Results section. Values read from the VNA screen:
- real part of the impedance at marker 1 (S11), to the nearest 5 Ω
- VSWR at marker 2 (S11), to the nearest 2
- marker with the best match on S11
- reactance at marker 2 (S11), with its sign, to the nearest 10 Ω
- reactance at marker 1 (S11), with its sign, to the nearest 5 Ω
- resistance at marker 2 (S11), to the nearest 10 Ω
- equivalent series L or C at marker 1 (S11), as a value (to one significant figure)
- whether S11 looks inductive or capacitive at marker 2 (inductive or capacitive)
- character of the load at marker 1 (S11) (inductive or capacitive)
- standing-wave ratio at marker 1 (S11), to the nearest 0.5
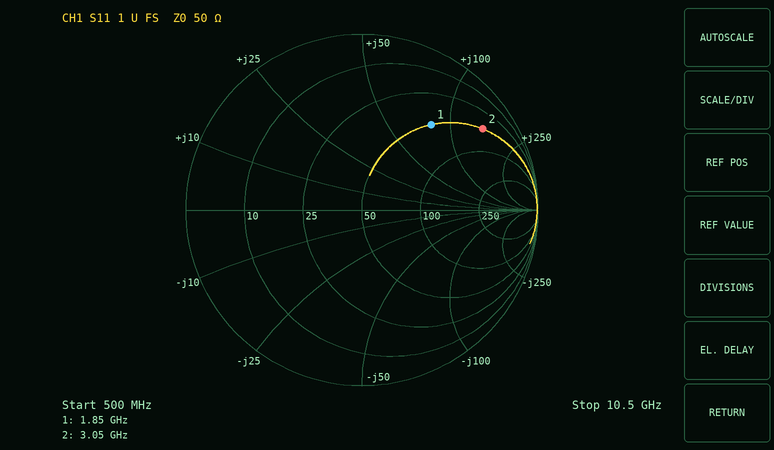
50 Ω
10
marker 1
+150 Ω
+80 Ω
50 Ω
7 nH
inductive
inductive
4.5
